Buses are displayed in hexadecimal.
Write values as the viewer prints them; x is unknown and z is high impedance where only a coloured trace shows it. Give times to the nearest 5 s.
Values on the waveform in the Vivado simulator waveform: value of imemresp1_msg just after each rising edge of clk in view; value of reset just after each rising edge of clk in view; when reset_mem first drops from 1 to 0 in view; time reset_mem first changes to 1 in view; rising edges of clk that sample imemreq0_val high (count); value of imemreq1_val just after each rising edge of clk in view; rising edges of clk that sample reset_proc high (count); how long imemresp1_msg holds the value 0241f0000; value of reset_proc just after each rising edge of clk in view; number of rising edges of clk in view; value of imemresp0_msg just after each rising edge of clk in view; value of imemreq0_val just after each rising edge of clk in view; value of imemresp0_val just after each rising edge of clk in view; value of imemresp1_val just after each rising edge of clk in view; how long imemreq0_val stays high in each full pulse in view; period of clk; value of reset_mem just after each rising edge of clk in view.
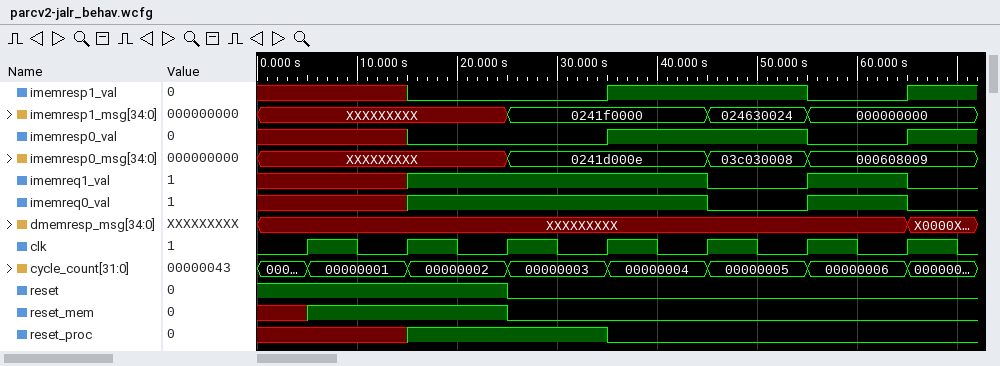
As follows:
XXXXXXXXX, XXXXXXXXX, 0241f0000, 0241f0000, 024630024, 000000000, 000000000
1 1 0 0 0 0 0
25 s
5 s
4
x 1 1 1 0 1 0
2
20 s
x 1 1 0 0 0 0
7
XXXXXXXXX, XXXXXXXXX, 0241d000e, 0241d000e, 03c030008, 000608009, 000608009
x 1 1 1 0 1 0
x 0 0 1 1 0 1
x 0 0 1 1 0 1
10 s
10 s
1 1 0 0 0 0 0
